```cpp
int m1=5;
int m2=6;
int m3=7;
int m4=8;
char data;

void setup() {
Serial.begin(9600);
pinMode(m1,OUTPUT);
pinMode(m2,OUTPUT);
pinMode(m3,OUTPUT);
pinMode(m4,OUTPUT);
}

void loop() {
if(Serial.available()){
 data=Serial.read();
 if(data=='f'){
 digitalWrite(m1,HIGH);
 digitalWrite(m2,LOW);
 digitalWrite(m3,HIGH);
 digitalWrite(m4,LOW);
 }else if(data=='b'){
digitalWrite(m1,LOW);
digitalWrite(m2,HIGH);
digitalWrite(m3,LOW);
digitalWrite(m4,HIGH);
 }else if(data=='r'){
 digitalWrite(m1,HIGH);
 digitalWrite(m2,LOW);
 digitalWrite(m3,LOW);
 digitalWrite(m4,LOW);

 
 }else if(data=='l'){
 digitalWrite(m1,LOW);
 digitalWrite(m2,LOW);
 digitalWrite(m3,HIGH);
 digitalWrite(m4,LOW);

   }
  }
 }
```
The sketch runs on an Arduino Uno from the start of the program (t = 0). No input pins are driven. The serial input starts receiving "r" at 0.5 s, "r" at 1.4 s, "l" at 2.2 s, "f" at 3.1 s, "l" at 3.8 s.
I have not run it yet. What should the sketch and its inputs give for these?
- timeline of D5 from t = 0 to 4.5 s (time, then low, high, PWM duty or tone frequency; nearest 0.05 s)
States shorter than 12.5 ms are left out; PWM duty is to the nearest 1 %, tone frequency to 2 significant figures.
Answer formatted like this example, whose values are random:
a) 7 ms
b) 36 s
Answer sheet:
a) 0 s low; 0.5 s high; 2.2 s low; 3.1 s high; 3.8 s low
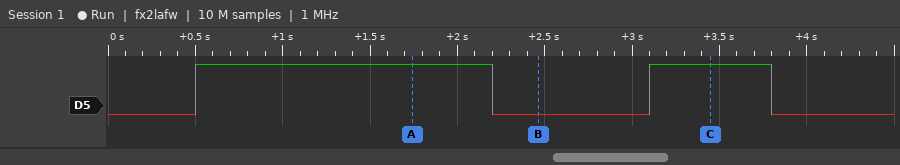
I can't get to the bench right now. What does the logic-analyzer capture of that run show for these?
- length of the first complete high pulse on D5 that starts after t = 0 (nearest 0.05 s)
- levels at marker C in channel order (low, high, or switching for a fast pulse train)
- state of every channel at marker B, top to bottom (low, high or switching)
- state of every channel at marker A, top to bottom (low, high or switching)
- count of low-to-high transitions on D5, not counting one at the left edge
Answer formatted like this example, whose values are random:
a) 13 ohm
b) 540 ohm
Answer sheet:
a) 1.70 s
b) D5 high
c) D5 low
d) D5 high
e) 2
